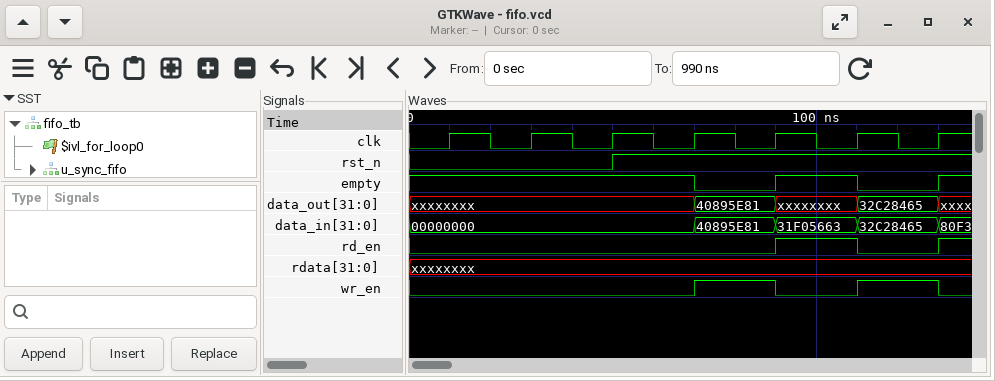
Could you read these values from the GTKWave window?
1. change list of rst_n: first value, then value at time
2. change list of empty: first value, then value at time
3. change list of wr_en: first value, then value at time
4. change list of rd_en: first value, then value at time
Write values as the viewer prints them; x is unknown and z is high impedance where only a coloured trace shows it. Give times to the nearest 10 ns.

0, 1 at 50 ns
1, 0 at 70 ns, 1 at 90 ns, 0 at 110 ns, 1 at 130 ns
0, 1 at 70 ns, 0 at 90 ns, 1 at 110 ns, 0 at 130 ns
0, 1 at 90 ns, 0 at 110 ns, 1 at 130 ns
